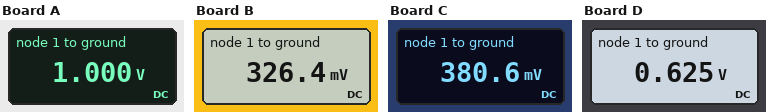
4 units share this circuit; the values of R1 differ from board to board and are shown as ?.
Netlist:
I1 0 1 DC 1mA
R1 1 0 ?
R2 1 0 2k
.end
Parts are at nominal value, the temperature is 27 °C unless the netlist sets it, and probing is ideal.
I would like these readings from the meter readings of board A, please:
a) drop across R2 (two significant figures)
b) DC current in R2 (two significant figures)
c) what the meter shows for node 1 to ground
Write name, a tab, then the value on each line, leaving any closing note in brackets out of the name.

drop across R2	1.0 V
DC current in R2	500 µA
what the meter shows for node 1 to ground	1.000 V
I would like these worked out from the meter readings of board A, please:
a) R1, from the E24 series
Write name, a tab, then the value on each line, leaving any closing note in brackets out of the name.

R1, from the E24 series	2 kΩ
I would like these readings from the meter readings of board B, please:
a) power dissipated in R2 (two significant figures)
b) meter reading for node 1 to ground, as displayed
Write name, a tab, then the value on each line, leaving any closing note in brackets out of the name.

power dissipated in R2	53 µW
meter reading for node 1 to ground, as displayed	326.4 mV
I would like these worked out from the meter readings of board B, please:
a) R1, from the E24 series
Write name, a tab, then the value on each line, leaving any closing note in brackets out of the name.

R1, from the E24 series	390 Ω
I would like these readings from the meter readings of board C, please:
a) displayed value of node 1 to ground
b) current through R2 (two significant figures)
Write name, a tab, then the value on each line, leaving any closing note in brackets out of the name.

displayed value of node 1 to ground	380.6 mV
current through R2	190 µA
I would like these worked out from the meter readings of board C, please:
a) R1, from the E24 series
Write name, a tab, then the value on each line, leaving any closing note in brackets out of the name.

R1, from the E24 series	470 Ω
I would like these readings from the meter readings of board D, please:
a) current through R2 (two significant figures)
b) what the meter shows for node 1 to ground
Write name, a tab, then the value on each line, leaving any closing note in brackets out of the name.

current through R2	310 µA
what the meter shows for node 1 to ground	0.625 V
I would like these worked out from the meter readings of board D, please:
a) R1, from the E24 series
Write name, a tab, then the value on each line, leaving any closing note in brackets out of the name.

R1, from the E24 series	910 Ω
